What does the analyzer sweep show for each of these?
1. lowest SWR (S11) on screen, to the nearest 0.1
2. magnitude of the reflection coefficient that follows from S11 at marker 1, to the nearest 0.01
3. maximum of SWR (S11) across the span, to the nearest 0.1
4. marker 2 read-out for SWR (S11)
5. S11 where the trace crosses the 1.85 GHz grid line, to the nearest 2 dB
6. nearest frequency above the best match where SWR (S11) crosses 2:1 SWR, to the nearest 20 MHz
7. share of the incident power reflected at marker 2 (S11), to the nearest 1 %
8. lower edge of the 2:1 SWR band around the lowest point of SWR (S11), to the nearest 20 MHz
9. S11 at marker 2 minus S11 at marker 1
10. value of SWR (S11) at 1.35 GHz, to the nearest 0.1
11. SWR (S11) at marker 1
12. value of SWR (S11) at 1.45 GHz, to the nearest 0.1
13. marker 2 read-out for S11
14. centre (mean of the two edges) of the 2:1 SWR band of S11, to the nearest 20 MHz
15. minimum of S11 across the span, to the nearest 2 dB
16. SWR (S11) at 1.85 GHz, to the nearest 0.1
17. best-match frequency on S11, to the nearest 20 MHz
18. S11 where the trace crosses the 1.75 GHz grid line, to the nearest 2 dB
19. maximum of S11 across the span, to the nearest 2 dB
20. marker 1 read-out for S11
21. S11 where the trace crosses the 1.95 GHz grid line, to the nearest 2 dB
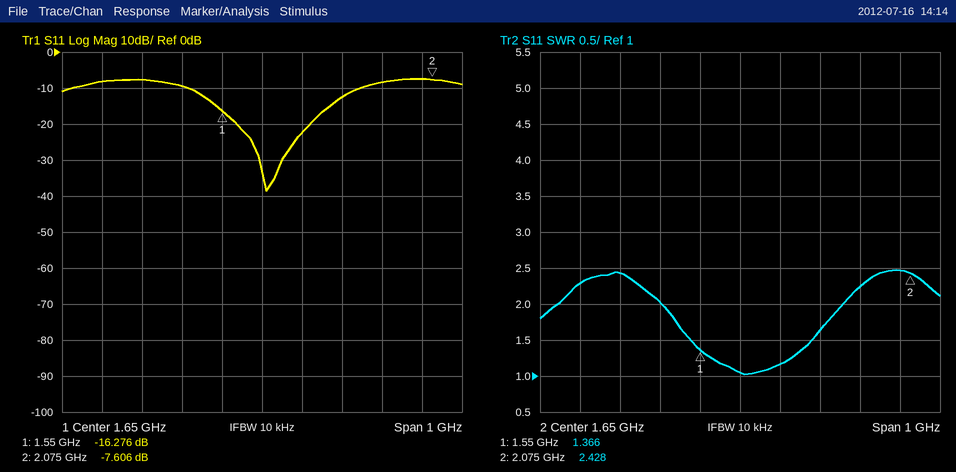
1.0
0.15
2.5
2.428
-12 dB
1.90 GHz
17 %
1.46 GHz
8.670 dB
2.4
1.366
2.0
-7.606 dB
1.68 GHz
-38 dB
1.6
1.66 GHz
-22 dB
-8 dB
-16.276 dB
-8 dB
